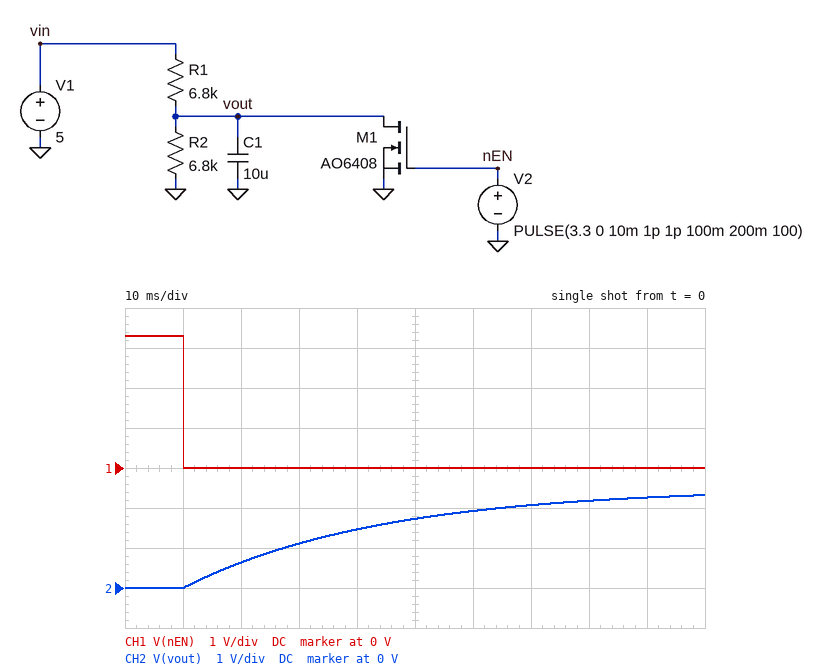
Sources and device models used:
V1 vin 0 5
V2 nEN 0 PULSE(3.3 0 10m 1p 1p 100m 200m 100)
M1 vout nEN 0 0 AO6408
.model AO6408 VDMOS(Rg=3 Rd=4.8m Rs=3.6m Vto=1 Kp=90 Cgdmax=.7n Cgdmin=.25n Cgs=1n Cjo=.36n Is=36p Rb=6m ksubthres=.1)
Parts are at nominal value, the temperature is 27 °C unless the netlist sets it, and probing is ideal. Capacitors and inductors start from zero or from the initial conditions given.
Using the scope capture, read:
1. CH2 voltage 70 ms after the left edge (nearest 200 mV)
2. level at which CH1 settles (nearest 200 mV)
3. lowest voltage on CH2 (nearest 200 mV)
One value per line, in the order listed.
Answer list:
2.0 V
0 V
0 V
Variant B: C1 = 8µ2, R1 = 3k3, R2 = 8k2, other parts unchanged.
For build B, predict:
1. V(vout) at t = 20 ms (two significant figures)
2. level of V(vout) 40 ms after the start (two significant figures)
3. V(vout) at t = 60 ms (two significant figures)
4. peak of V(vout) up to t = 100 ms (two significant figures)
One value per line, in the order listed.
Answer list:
1.4 V
2.8 V
3.3 V
3.5 V
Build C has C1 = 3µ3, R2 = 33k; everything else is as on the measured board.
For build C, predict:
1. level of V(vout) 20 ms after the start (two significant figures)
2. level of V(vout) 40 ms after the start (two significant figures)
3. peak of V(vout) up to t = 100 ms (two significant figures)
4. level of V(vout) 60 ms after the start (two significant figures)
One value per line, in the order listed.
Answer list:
1.7 V
3.3 V
4.1 V
3.9 V
